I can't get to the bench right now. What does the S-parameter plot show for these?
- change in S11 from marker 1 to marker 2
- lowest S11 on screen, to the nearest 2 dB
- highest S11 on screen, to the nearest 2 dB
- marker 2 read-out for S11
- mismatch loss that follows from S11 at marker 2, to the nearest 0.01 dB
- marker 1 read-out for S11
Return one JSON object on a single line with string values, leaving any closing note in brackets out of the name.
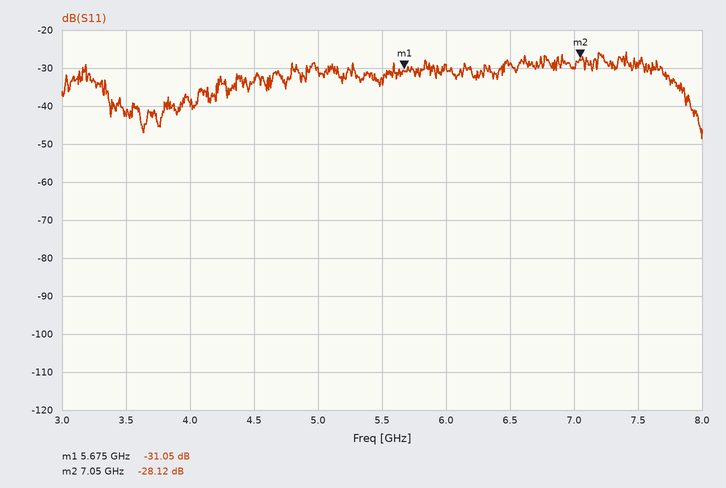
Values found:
{"change in S11 from marker 1 to marker 2": "2.93 dB", "lowest S11 on screen, to the nearest 2 dB": "-48 dB", "highest S11 on screen, to the nearest 2 dB": "-26 dB", "marker 2 read-out for S11": "-28.12 dB", "mismatch loss that follows from S11 at marker 2, to the nearest 0.01 dB": "0.01 dB", "marker 1 read-out for S11": "-31.05 dB"}
